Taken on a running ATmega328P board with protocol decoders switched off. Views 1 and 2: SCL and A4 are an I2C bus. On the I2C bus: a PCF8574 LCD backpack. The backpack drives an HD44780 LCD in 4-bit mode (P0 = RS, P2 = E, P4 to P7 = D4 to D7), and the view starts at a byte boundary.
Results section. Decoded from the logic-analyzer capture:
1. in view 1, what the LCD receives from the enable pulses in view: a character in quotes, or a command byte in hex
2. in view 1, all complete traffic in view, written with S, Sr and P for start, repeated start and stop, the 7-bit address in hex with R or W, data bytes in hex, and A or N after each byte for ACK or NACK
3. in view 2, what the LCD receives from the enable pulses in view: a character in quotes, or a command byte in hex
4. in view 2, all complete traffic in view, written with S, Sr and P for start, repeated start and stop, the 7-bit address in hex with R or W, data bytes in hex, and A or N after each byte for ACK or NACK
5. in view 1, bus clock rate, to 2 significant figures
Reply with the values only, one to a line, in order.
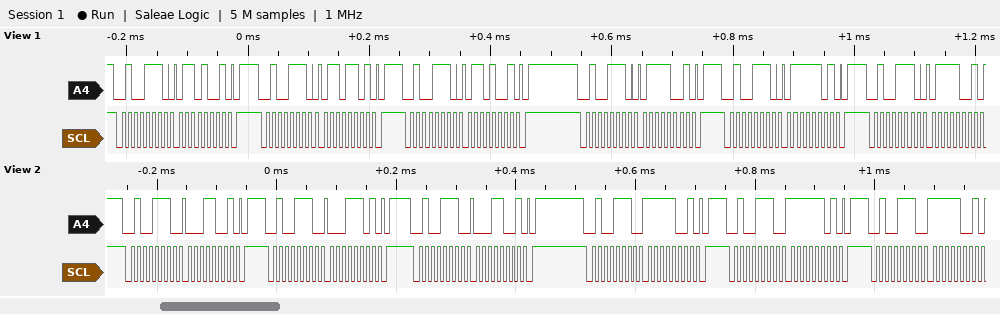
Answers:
'g'
S 27W A 69 A P S 27W A 6D A P S 27W A 69 A P S 27W A 79 A P S 27W A 7D A P S 27W A 79 A
data 0x1F
S 27W A 19 A P S 27W A 1D A P S 27W A 19 A P S 27W A F9 A P S 27W A FD A P S 27W A F9 A
100 kHz
